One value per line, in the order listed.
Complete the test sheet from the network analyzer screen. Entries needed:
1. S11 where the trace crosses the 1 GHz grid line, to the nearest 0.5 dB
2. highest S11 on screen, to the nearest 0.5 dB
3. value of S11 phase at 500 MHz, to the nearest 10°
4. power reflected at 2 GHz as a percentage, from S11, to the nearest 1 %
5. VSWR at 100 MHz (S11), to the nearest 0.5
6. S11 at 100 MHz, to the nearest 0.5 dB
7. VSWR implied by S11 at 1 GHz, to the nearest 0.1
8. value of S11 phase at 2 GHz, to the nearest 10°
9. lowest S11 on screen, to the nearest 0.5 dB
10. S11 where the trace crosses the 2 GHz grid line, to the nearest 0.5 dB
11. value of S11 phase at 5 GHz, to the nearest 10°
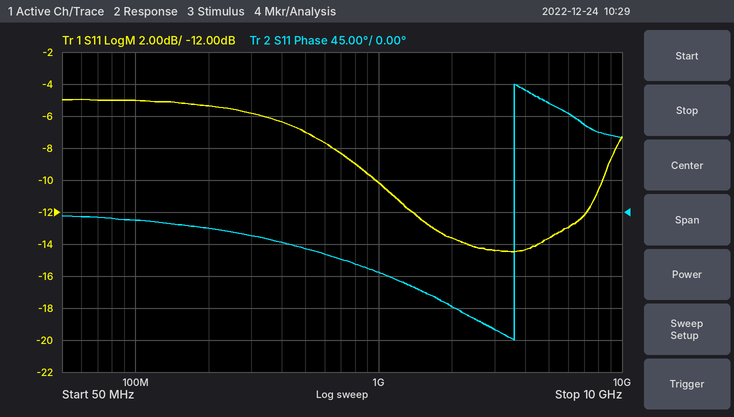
-10.0 dB
-5.0 dB
-50°
4 %
3.5
-5.0 dB
1.9
-130°
-14.5 dB
-13.5 dB
150°
